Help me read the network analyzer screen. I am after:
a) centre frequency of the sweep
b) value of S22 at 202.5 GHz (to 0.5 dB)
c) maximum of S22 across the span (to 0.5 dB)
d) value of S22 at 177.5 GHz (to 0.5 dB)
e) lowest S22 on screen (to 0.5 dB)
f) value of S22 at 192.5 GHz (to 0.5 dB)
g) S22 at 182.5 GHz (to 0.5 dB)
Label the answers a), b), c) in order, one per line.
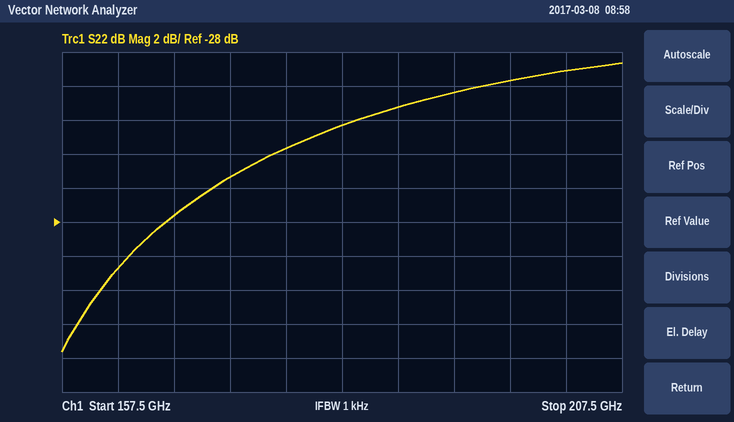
a) 182.5 GHz
b) -19.0 dB
c) -18.5 dB
d) -23.5 dB
e) -35.5 dB
f) -20.5 dB
g) -22.5 dB
